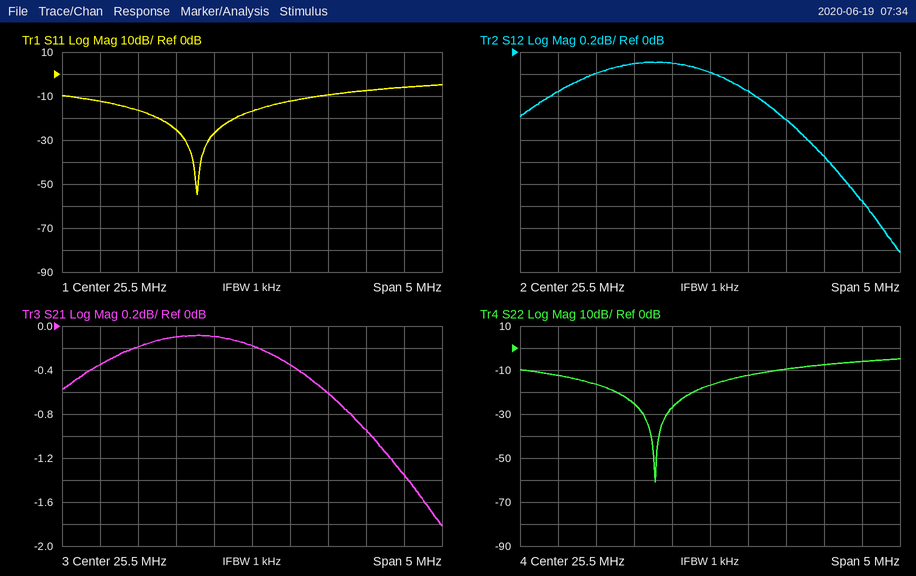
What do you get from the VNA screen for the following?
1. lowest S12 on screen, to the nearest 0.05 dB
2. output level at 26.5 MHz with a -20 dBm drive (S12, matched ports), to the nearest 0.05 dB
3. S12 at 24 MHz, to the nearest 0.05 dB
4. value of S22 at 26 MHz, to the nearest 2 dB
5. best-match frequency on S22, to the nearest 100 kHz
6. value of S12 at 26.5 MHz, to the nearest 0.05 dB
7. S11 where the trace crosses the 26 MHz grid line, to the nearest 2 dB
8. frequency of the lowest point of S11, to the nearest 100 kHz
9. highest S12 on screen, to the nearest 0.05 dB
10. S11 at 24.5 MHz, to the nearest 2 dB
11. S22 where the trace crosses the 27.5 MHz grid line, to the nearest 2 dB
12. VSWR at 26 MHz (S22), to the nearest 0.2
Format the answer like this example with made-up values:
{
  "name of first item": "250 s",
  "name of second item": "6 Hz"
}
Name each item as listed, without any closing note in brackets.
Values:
{
  "lowest S12 on screen, to the nearest 0.05 dB": "-1.80 dB",
  "output level at 26.5 MHz with a -20 dBm drive (S12, matched ports), to the nearest 0.05 dB": "-20.60 dBm",
  "S12 at 24 MHz, to the nearest 0.05 dB": "-0.20 dB",
  "value of S22 at 26 MHz, to the nearest 2 dB": "-12 dB",
  "best-match frequency on S22, to the nearest 100 kHz": "24.8 MHz",
  "value of S12 at 26.5 MHz, to the nearest 0.05 dB": "-0.60 dB",
  "S11 where the trace crosses the 26 MHz grid line, to the nearest 2 dB": "-12 dB",
  "frequency of the lowest point of S11, to the nearest 100 kHz": "24.8 MHz",
  "highest S12 on screen, to the nearest 0.05 dB": "-0.10 dB",
  "S11 at 24.5 MHz, to the nearest 2 dB": "-26 dB",
  "S22 where the trace crosses the 27.5 MHz grid line, to the nearest 2 dB": "-6 dB",
  "VSWR at 26 MHz (S22), to the nearest 0.2": "1.6"
}
